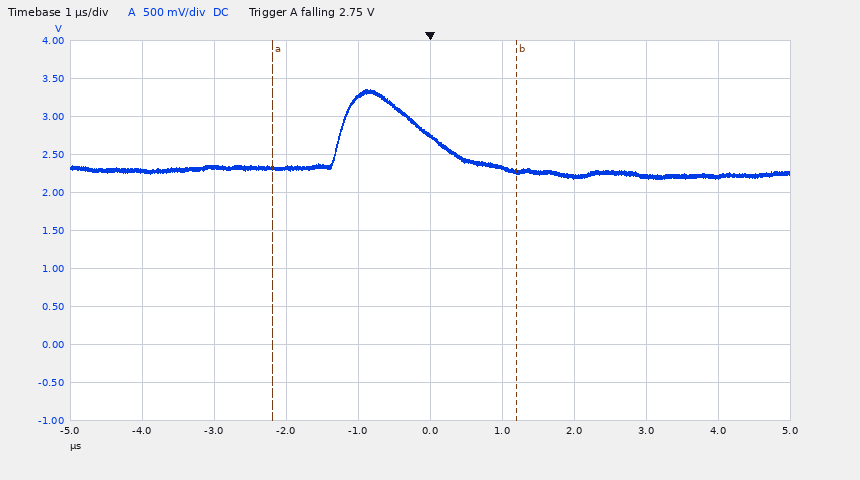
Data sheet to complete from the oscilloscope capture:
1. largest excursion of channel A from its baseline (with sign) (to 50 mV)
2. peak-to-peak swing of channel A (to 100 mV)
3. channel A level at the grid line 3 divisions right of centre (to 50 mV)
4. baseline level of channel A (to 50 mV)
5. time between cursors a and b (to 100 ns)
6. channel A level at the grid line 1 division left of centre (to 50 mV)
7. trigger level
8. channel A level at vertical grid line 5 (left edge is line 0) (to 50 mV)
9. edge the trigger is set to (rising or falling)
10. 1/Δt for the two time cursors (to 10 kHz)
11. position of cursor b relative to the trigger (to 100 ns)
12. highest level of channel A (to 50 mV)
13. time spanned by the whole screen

+1.05 V
1.20 V
2.20 V
2.30 V
3.4 µs
3.25 V
2.75 V
2.75 V
falling
290 kHz
+1.2 µs
3.35 V
10 µs
